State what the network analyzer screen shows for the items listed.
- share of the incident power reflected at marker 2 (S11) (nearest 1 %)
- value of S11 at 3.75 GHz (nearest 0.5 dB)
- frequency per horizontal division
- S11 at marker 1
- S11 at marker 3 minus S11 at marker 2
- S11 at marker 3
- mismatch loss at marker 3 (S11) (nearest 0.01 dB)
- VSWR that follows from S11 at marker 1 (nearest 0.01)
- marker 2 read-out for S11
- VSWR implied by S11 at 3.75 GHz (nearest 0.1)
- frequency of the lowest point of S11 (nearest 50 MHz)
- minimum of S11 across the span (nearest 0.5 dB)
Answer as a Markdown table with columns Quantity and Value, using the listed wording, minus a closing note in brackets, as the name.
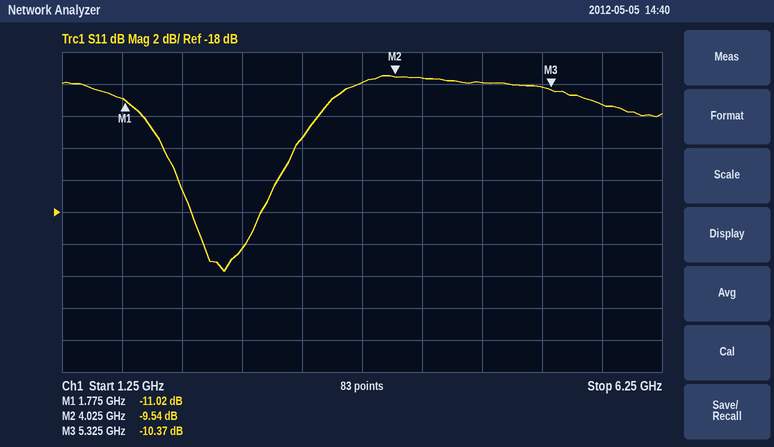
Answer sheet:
| Quantity | Value |
|---|---|
| share of the incident power reflected at marker 2 (S11) | 11 % |
| value of S11 at 3.75 GHz | -10.0 dB |
| frequency per horizontal division | 500 MHz |
| S11 at marker 1 | -11.02 dB |
| S11 at marker 3 minus S11 at marker 2 | -0.83 dB |
| S11 at marker 3 | -10.37 dB |
| mismatch loss at marker 3 (S11) | 0.42 dB |
| VSWR that follows from S11 at marker 1 | 1.78 |
| marker 2 read-out for S11 | -9.54 dB |
| VSWR implied by S11 at 3.75 GHz | 1.9 |
| frequency of the lowest point of S11 | 2.60 GHz |
| minimum of S11 across the span | -21.5 dB |
